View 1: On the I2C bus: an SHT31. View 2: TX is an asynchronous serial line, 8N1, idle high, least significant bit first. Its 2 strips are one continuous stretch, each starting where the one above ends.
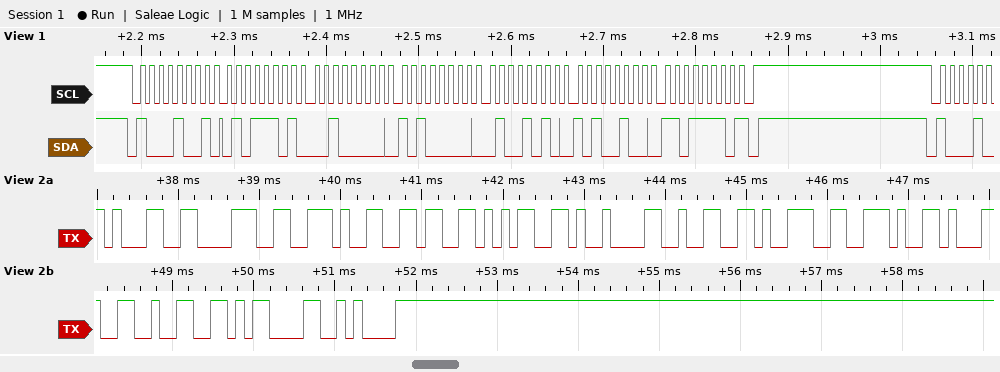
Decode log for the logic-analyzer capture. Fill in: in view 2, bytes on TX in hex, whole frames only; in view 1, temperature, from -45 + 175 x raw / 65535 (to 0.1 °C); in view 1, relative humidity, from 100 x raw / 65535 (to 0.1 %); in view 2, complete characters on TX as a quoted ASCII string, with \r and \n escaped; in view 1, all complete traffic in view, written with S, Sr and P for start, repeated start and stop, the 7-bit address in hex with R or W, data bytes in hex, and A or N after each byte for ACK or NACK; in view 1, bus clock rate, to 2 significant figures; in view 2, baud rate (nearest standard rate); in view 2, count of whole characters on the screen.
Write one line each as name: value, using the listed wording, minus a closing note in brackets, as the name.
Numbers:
in view 2, bytes on TX in hex, whole frames only: 31 38 2E 36 35 09 32 39 2E 31 32 0D 0A
in view 1, temperature, from -45 + 175 x raw / 65535: 18.7 °C
in view 1, relative humidity, from 100 x raw / 65535: 29.2 %
in view 2, complete characters on TX as a quoted ASCII string, with \r and \n escaped: "18.65\t29.12\r\n"
in view 1, all complete traffic in view, written with S, Sr and P for start, repeated start and stop, the 7-bit address in hex with R or W, data bytes in hex, and A or N after each byte for ACK or NACK: S 44R A 5D A 20 A A0 A 4A A A4 A DE N P
in view 1, bus clock rate, to 2 significant figures: 100 kHz
in view 2, baud rate: 9600 baud
in view 2, count of whole characters on the screen: 13
